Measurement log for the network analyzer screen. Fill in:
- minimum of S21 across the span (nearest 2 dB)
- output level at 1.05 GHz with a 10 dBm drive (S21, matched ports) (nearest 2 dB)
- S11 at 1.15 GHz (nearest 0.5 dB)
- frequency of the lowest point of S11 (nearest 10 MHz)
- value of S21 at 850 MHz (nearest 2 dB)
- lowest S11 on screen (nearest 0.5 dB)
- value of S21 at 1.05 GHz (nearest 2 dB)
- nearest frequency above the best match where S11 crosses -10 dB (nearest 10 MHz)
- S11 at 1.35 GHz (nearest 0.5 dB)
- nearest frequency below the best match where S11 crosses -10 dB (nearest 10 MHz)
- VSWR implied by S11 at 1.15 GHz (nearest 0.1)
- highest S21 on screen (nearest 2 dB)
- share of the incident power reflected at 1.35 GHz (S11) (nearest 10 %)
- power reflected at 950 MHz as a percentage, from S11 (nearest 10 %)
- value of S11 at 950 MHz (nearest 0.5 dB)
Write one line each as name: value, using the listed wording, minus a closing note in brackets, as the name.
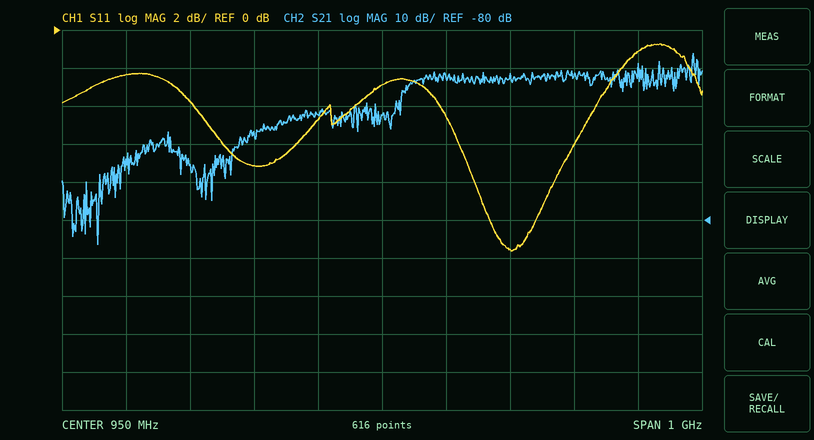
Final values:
minimum of S21 across the span: -86 dB
output level at 1.05 GHz with a 10 dBm drive (S21, matched ports): -32 dBm
S11 at 1.15 GHz: -11.5 dB
frequency of the lowest point of S11: 1.15 GHz
value of S21 at 850 MHz: -52 dB
lowest S11 on screen: -11.5 dB
value of S21 at 1.05 GHz: -42 dB
nearest frequency above the best match where S11 crosses -10 dB: 1.19 GHz
S11 at 1.35 GHz: -1.0 dB
nearest frequency below the best match where S11 crosses -10 dB: 1.12 GHz
VSWR implied by S11 at 1.15 GHz: 1.7
highest S21 on screen: -36 dB
share of the incident power reflected at 1.35 GHz (S11): 80 %
power reflected at 950 MHz as a percentage, from S11: 50 %
value of S11 at 950 MHz: -3.0 dB
